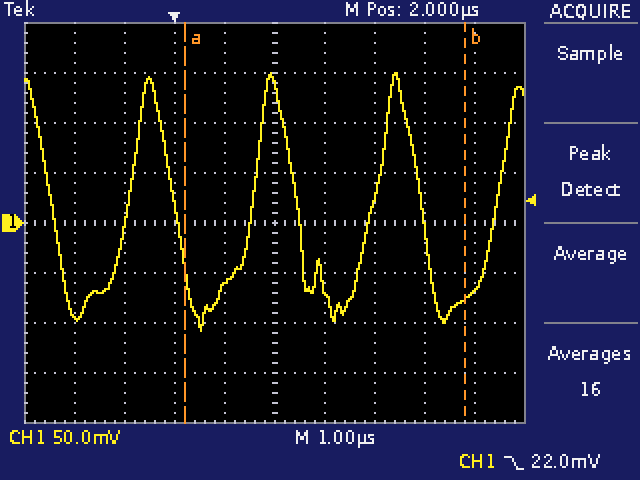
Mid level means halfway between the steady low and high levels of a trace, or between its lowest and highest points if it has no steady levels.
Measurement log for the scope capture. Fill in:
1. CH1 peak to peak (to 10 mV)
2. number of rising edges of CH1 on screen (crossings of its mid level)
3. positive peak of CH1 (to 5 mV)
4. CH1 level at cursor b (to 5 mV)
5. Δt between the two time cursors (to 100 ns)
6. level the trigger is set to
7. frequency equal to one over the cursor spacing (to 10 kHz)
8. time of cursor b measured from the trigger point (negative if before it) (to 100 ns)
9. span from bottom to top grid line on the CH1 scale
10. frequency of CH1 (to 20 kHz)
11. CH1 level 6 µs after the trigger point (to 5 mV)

260 mV
4
150 mV
-75 mV
5.6 µs
22.0 mV
180 kHz
+5.8 µs
400 mV
400 kHz
-70 mV
